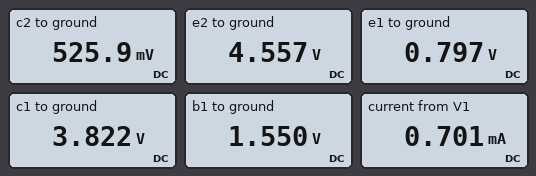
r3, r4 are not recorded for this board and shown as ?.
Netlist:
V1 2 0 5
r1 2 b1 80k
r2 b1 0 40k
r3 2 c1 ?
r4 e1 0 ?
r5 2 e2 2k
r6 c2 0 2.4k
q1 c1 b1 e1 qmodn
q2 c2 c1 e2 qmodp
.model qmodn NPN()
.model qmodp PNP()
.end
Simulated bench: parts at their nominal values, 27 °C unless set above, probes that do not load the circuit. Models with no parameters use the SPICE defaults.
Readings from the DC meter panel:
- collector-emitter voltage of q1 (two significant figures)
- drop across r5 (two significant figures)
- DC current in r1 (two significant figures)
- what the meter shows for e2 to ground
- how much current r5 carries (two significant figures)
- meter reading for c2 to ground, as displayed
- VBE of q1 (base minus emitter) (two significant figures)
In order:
3.0 V
440 mV
43 µA
4.557 V
220 µA
525.9 mV
750 mV
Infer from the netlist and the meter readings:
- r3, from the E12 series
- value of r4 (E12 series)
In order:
2.7 kΩ
1.8 kΩ
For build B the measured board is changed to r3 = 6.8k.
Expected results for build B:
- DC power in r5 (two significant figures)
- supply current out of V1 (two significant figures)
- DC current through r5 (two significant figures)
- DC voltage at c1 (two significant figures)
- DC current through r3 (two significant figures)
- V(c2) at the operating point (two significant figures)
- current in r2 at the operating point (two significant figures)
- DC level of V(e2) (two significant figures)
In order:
2.3 mW
1.5 mA
1.1 mA
2.1 V
430 µA
2.5 V
39 µA
2.9 V
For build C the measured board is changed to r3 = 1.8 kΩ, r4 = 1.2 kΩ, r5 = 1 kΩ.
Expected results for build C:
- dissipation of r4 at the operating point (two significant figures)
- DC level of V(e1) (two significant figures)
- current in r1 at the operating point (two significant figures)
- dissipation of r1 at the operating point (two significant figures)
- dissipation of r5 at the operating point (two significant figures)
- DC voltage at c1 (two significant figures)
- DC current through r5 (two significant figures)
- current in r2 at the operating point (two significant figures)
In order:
460 µW
740 mV
44 µA
150 µW
120 µW
3.9 V
350 µA
38 µA
